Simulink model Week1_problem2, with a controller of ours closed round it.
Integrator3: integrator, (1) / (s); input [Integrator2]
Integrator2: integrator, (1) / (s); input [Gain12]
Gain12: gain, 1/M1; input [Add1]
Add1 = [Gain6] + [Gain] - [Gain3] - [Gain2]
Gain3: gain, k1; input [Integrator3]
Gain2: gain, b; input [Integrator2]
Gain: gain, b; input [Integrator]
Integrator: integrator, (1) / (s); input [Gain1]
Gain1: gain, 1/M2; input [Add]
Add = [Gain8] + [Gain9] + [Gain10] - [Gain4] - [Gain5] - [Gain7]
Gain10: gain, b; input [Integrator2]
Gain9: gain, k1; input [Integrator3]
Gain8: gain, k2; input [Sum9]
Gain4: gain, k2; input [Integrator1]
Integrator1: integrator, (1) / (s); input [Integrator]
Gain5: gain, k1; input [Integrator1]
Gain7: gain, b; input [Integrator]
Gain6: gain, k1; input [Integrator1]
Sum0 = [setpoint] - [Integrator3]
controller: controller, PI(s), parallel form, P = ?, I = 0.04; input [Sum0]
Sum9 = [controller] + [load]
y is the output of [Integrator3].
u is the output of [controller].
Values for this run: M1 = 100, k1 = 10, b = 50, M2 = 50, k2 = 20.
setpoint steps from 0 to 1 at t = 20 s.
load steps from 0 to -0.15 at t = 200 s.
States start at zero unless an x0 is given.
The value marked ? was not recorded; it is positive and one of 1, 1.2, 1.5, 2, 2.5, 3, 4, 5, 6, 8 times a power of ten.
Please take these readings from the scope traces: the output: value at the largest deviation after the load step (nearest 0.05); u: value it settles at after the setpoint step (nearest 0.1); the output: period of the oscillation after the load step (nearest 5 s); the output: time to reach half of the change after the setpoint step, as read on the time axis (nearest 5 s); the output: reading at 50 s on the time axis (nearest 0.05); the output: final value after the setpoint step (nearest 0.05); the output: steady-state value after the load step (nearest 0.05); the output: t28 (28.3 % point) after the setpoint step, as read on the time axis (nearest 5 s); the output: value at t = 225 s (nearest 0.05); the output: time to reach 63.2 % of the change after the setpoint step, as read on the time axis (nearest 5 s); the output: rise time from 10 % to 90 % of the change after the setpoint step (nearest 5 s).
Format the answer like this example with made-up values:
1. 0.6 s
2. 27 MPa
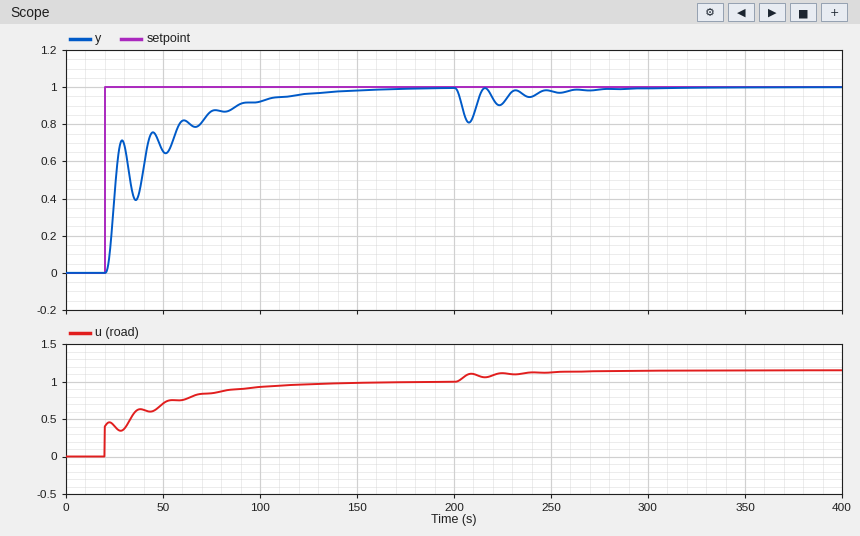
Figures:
1. 0.80
2. 1.0
3. 15 s
4. 25 s
5. 0.65
6. 1.00
7. 1.00
8. 25 s
9. 0.90
10. 25 s
11. 65 s
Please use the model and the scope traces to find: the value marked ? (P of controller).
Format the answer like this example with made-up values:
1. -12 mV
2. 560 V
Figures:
1. 0.4
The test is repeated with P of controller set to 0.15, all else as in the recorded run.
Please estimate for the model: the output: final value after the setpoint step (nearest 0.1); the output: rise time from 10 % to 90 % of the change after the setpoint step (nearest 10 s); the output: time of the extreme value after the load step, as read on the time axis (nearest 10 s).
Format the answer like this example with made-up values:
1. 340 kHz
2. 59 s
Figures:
1. 1.0
2. 60 s
3. 210 s
